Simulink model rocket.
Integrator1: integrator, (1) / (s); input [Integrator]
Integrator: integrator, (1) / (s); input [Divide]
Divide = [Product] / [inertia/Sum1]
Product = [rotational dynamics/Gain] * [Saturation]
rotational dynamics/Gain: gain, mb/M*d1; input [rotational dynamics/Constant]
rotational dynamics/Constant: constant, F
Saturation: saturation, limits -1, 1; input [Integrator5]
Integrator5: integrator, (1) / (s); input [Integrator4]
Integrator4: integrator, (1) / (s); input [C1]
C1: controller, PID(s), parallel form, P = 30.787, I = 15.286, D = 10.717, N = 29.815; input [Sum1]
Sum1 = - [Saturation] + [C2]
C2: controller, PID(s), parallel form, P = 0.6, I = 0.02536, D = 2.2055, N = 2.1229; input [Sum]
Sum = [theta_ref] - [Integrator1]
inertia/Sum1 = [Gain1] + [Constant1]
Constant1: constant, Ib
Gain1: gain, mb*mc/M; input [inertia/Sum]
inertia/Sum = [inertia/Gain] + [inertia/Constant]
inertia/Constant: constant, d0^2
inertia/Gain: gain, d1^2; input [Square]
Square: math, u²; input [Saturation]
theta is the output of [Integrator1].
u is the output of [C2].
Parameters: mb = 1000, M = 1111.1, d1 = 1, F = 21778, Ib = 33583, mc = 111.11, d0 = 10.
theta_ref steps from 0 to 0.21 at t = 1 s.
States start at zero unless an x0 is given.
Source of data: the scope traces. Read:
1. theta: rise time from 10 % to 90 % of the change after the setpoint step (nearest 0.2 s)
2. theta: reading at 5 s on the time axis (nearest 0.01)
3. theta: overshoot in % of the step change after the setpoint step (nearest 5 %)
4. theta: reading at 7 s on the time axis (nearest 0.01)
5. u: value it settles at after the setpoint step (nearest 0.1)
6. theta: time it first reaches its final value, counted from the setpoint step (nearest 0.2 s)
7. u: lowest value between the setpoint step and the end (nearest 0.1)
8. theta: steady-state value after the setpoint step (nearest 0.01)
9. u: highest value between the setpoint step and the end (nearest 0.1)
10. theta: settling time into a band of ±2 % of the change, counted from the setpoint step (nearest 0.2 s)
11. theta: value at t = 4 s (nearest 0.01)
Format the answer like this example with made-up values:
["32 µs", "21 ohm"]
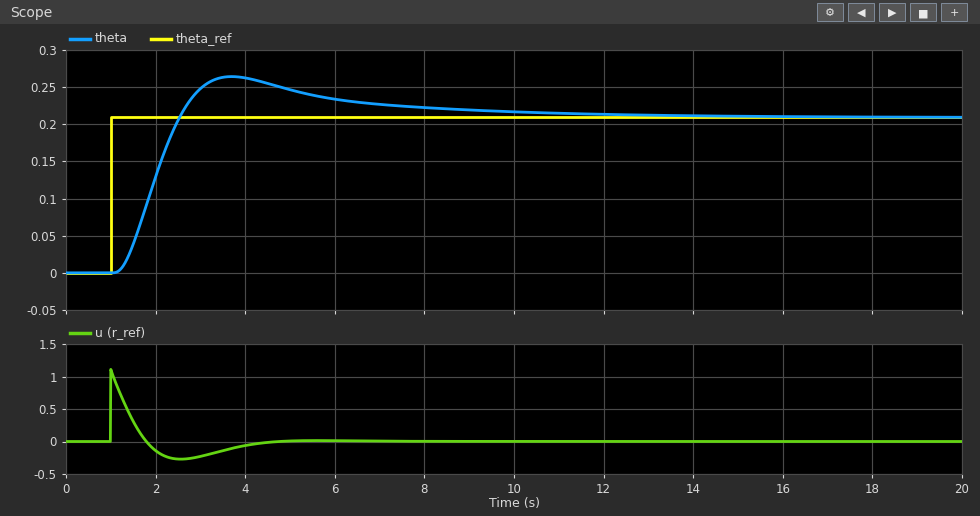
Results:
["1.0 s", "0.25", "25 %", "0.23", "0.0", "1.6 s", "-0.3", "0.21", "1.1", "10.4 s", "0.26"]
